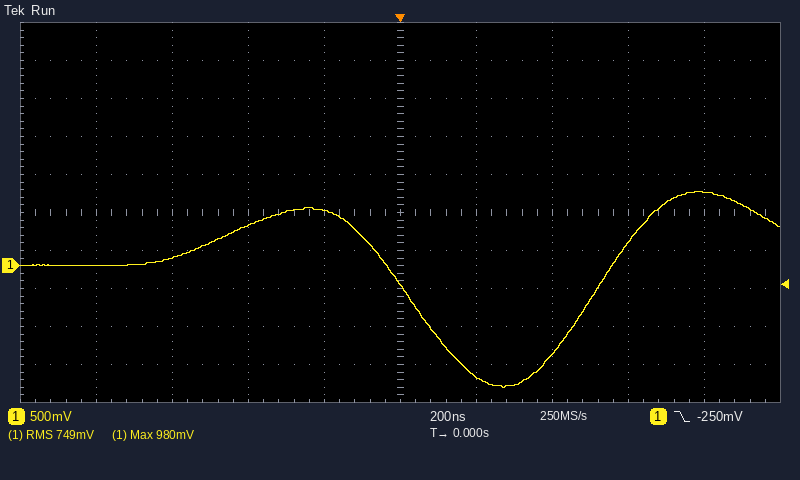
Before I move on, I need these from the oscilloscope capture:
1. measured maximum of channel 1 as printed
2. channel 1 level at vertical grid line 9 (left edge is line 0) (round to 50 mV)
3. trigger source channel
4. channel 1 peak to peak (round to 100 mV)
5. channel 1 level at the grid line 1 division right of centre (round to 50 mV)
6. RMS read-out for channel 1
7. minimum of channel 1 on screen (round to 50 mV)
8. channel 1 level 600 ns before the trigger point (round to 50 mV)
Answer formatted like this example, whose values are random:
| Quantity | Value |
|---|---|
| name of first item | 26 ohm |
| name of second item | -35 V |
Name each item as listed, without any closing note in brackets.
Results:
| Quantity | Value |
|---|---|
| measured maximum of channel 1 as printed | 980 mV |
| channel 1 level at vertical grid line 9 (left edge is line 0) | 950 mV |
| trigger source channel | channel 1 |
| channel 1 peak to peak | 2.60 V |
| channel 1 level at the grid line 1 division right of centre | -1.45 V |
| RMS read-out for channel 1 | 749 mV |
| minimum of channel 1 on screen | -1.60 V |
| channel 1 level 600 ns before the trigger point | 100 mV |
